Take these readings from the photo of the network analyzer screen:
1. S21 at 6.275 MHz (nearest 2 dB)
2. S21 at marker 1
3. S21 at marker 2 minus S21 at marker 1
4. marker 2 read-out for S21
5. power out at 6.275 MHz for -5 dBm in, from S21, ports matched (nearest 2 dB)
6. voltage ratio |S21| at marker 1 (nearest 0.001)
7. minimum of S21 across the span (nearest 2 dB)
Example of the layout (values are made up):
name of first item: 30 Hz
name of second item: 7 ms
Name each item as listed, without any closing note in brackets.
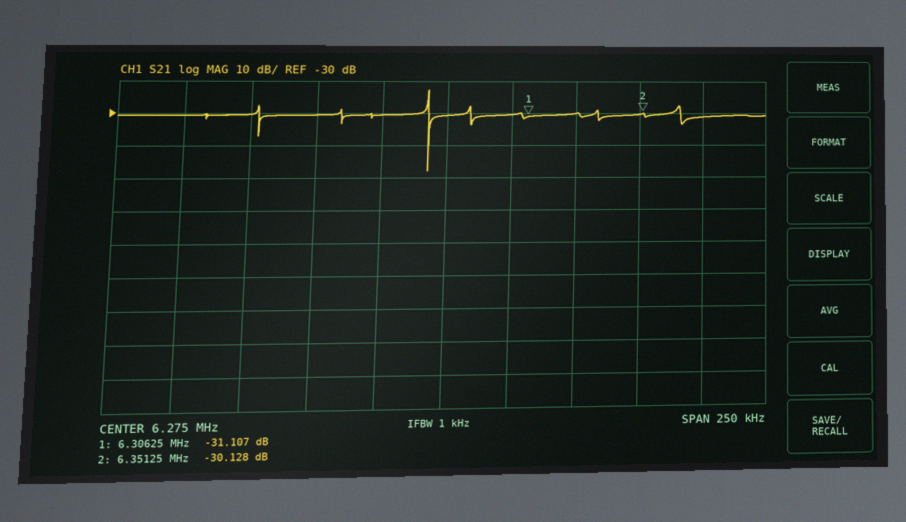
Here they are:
S21 at 6.275 MHz: -30 dB
S21 at marker 1: -31.107 dB
S21 at marker 2 minus S21 at marker 1: 0.979 dB
marker 2 read-out for S21: -30.128 dB
power out at 6.275 MHz for -5 dBm in, from S21, ports matched: -36 dBm
voltage ratio |S21| at marker 1: 0.028
minimum of S21 across the span: -48 dB
